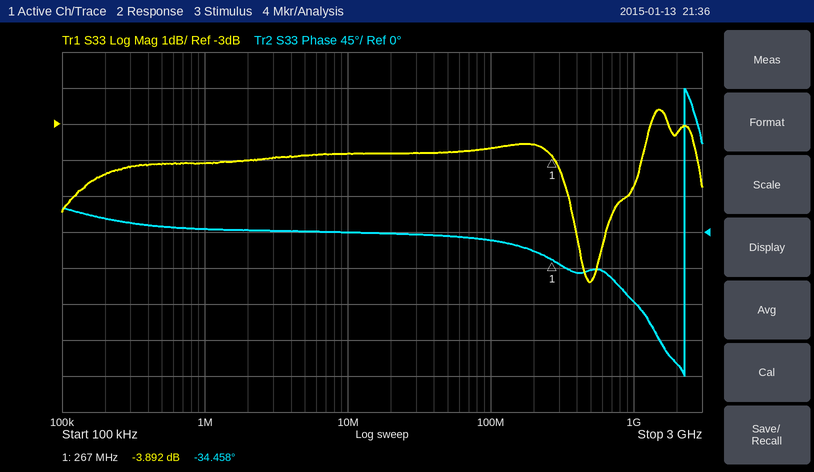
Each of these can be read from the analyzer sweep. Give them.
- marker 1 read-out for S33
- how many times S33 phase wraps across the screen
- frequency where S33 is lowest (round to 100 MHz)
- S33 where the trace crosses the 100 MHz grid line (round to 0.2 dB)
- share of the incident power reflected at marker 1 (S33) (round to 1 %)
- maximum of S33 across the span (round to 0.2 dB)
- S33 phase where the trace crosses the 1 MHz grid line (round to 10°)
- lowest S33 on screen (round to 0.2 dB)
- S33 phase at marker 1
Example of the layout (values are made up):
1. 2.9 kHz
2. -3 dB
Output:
1. -3.892 dB
2. 1
3. 500 MHz
4. -3.6 dB
5. 41 %
6. -2.6 dB
7. 0°
8. -7.4 dB
9. -34.458°
